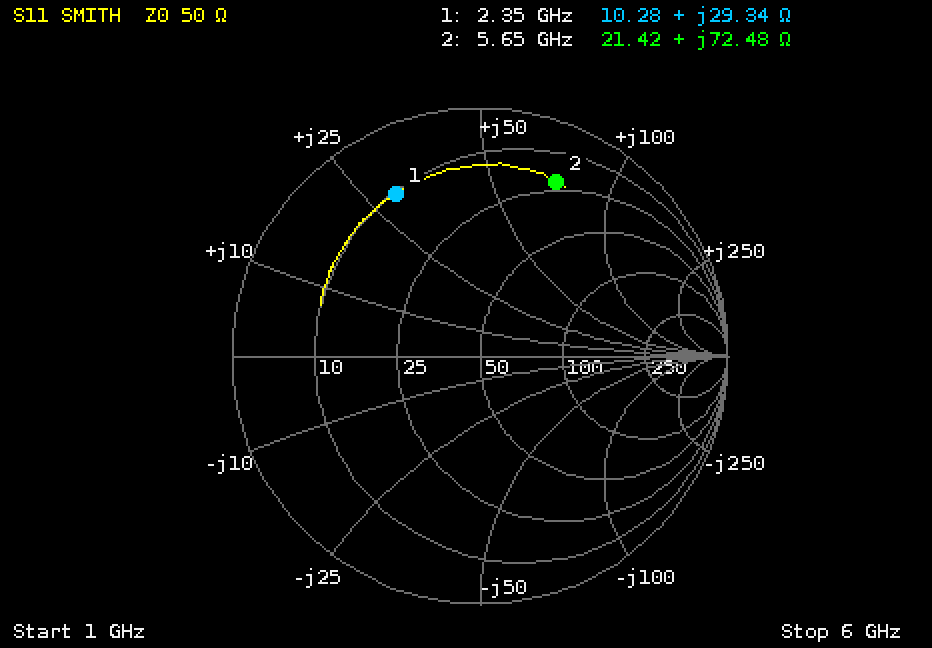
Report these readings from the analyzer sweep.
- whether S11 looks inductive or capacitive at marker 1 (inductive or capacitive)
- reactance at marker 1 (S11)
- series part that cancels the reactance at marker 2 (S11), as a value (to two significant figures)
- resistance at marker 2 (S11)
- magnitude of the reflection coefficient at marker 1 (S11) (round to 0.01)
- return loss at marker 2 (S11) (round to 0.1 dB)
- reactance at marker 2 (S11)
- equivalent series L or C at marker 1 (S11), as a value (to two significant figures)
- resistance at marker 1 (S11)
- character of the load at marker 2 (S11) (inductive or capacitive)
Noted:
inductive
+29.34 Ω
390 fF
21.42 Ω
0.74
2.3 dB
+72.48 Ω
2.0 nH
10.28 Ω
inductive
